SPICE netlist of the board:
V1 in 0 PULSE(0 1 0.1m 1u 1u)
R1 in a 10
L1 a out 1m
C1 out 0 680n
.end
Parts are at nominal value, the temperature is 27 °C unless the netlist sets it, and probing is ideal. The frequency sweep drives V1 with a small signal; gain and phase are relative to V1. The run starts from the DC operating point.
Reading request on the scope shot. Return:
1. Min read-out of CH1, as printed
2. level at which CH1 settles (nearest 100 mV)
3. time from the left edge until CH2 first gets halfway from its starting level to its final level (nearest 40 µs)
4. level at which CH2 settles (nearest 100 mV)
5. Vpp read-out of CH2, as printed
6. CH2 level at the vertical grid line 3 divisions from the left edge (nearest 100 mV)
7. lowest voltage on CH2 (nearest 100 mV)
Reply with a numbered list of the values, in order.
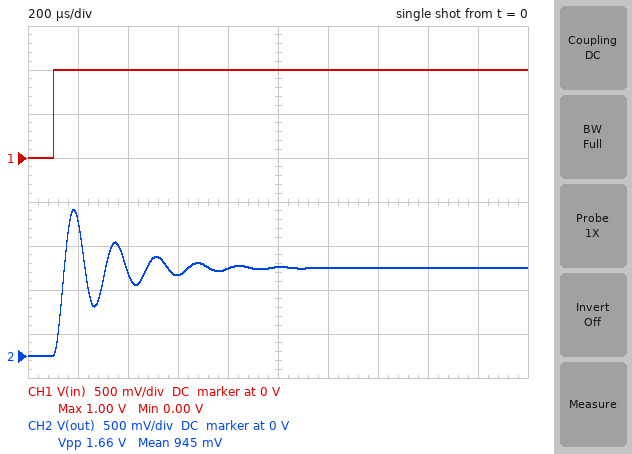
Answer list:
1. 0.00 V
2. 1.0 V
3. 120 µs
4. 1.0 V
5. 1.66 V
6. 900 mV
7. 0 V
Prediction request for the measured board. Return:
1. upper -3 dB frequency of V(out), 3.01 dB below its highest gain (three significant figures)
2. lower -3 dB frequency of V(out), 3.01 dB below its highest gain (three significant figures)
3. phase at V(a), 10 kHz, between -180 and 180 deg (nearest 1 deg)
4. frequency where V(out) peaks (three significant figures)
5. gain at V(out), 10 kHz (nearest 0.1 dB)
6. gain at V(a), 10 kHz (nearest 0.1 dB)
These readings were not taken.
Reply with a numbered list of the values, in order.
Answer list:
1. 6.75 kHz
2. 5.13 kHz
3. 14 deg
4. 6.00 kHz
5. -4.8 dB
6. -0.3 dB
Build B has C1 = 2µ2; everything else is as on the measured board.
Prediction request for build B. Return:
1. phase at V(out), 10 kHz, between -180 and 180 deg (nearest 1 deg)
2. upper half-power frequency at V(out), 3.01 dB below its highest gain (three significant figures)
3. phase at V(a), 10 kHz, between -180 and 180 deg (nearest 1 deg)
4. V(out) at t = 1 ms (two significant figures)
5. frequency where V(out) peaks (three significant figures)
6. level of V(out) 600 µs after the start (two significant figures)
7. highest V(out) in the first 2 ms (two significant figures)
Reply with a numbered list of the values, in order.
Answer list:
1. -170 deg
2. 3.94 kHz
3. 10 deg
4. 990 mV
5. 3.20 kHz
6. 1.1 V
7. 1.5 V
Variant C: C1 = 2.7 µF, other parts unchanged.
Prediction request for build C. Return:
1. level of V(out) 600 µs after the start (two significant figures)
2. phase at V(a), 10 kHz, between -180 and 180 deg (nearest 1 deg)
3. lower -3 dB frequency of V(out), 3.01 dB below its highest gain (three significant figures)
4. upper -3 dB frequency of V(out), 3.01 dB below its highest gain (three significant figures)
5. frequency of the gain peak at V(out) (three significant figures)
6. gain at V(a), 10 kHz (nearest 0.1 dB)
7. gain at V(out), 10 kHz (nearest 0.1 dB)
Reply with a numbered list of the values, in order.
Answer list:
1. 1.1 V
2. 10 deg
3. 1.85 kHz
4. 3.58 kHz
5. 2.85 kHz
6. -0.1 dB
7. -19.8 dB
